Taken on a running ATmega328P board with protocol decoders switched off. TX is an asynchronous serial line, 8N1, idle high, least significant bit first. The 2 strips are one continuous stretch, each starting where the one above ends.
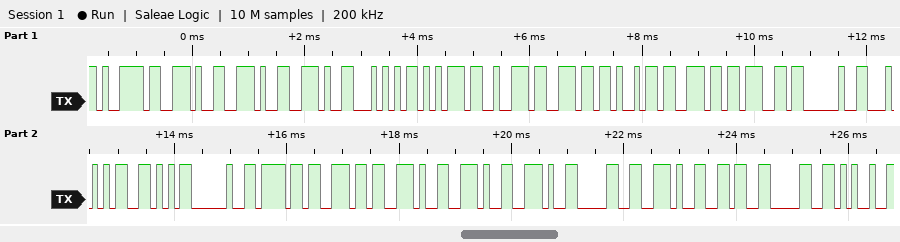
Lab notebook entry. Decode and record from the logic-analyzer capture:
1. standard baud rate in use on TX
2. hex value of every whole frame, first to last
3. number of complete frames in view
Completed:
9600 baud
79 2E 2E 2E 54 75 72 6E 69 6E 67 20 54 56 20 6F 6E 2E 2E 2E 30 2E 36 30 25
25
